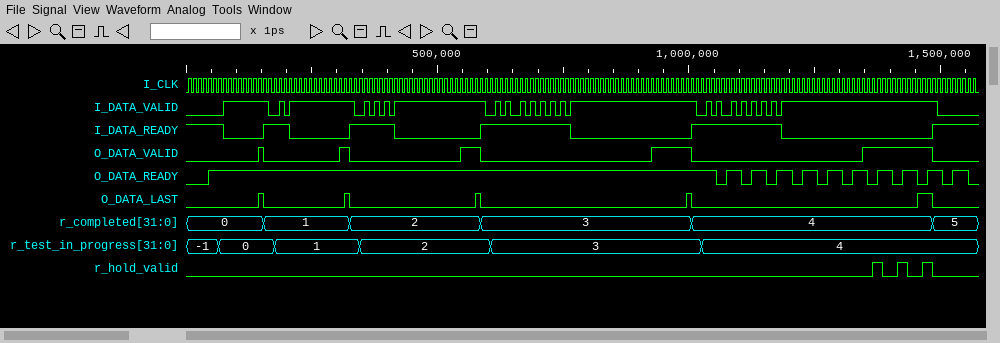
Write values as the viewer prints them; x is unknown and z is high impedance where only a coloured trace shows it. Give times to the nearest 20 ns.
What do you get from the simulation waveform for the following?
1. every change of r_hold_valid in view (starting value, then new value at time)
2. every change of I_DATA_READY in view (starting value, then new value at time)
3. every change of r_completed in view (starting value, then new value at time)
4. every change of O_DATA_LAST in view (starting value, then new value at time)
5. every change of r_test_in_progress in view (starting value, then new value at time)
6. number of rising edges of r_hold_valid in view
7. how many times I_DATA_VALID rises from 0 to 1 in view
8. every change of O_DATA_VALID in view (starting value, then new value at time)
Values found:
0, 1 at 1360 ns, 0 at 1380 ns, 1 at 1420 ns, 0 at 1440 ns, 1 at 1460 ns, 0 at 1480 ns
1, 0 at 80 ns, 1 at 160 ns, 0 at 200 ns, 1 at 320 ns, 0 at 420 ns, 1 at 580 ns, 0 at 760 ns, 1 at 1000 ns, 0 at 1180 ns, 1 at 1480 ns
0, 1 at 160 ns, 2 at 320 ns, 3 at 580 ns, 4 at 1000 ns, 5 at 1480 ns
0, 1 at 140 ns, 0 at 160 ns, 1 at 320 ns, 0 at 320 ns, 1 at 580 ns, 0 at 580 ns, 1 at 1000 ns, 0 at 1000 ns, 1 at 1460 ns, 0 at 1480 ns
-1, 0 at 60 ns, 1 at 180 ns, 2 at 340 ns, 3 at 600 ns, 4 at 1020 ns
3
23
0, 1 at 140 ns, 0 at 160 ns, 1 at 300 ns, 0 at 320 ns, 1 at 540 ns, 0 at 580 ns, 1 at 920 ns, 0 at 1000 ns, 1 at 1340 ns, 0 at 1480 ns
